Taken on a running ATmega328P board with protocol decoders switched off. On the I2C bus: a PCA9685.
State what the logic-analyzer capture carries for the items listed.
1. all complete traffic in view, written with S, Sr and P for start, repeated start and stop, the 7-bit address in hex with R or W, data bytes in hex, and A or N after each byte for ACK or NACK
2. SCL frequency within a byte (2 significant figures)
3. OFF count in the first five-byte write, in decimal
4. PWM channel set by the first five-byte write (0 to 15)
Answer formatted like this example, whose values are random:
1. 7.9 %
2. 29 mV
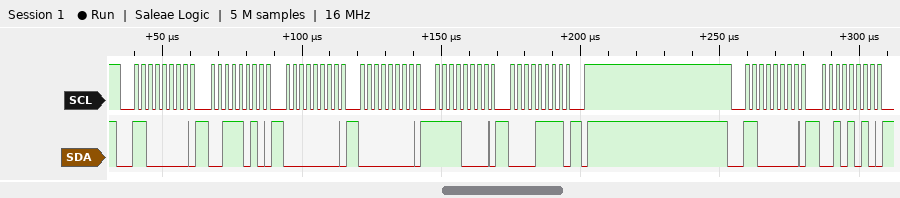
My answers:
1. S 60W A 3A A 00 A 00 A F0 A 0F A P S 60W A 2A A
2. 400 kHz
3. 4080
4. 13
